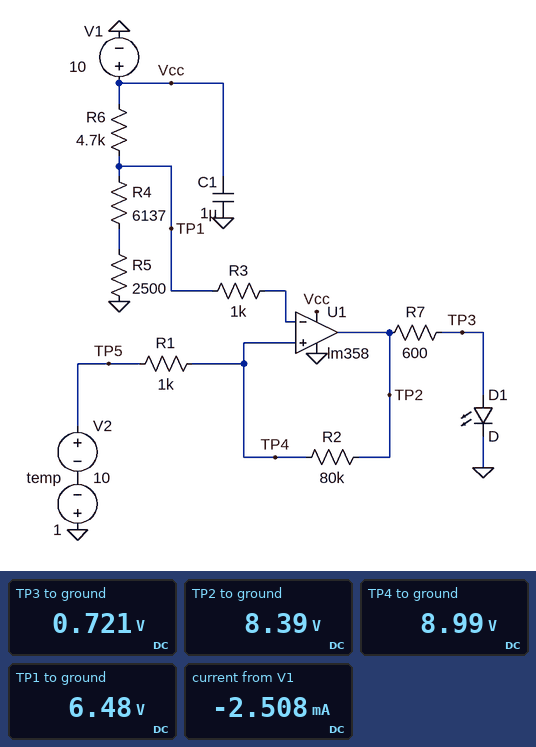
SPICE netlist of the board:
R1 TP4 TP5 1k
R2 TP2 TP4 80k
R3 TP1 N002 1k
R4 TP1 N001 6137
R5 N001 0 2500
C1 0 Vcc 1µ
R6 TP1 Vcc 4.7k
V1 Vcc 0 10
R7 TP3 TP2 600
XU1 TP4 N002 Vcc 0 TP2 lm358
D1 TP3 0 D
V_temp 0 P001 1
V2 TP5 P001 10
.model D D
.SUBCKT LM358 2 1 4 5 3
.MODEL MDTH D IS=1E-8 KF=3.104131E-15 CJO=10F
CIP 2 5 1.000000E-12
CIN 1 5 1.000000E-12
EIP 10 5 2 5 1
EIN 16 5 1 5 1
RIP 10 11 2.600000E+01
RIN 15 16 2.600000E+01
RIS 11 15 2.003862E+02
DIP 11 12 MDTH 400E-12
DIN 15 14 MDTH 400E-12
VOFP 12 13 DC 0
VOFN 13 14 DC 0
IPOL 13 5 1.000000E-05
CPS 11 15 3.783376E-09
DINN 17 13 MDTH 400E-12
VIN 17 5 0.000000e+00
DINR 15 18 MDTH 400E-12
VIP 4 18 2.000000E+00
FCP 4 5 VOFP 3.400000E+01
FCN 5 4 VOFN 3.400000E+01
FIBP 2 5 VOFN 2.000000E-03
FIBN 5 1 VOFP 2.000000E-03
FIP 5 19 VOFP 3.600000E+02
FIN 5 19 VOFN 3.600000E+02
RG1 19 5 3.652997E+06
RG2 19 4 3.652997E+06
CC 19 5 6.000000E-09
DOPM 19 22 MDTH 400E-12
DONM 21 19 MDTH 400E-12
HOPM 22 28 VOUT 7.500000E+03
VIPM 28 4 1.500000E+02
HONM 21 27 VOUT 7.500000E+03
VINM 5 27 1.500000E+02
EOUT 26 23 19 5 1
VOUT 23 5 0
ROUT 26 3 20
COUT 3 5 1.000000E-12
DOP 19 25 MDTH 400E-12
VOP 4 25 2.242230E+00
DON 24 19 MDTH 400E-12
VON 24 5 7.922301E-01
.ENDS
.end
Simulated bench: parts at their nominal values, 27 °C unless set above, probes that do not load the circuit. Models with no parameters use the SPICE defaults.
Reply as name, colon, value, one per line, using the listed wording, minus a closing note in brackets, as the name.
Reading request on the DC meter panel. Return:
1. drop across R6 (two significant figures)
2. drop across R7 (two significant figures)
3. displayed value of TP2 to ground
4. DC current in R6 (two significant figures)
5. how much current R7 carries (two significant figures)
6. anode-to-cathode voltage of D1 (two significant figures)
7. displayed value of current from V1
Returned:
drop across R6: 3.5 V
drop across R7: 7.7 V
displayed value of TP2 to ground: 8.39 V
DC current in R6: 750 µA
how much current R7 carries: 13 mA
anode-to-cathode voltage of D1: 720 mV
displayed value of current from V1: -2.508 mA
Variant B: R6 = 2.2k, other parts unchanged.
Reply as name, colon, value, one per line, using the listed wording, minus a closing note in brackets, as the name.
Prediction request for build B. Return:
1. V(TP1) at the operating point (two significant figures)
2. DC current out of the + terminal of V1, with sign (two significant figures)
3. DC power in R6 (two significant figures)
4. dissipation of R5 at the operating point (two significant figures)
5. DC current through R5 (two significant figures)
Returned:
V(TP1) at the operating point: 8.0 V
DC current out of the + terminal of V1, with sign: -2.3 mA
DC power in R6: 1.9 mW
dissipation of R5 at the operating point: 2.1 mW
DC current through R5: 920 µA
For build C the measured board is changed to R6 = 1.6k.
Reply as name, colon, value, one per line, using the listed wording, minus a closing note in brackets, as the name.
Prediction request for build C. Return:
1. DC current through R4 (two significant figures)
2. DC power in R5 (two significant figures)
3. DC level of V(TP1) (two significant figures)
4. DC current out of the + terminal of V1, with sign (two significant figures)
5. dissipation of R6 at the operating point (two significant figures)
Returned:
DC current through R4: 980 µA
DC power in R5: 2.4 mW
DC level of V(TP1): 8.4 V
DC current out of the + terminal of V1, with sign: -2.3 mA
dissipation of R6 at the operating point: 1.5 mW
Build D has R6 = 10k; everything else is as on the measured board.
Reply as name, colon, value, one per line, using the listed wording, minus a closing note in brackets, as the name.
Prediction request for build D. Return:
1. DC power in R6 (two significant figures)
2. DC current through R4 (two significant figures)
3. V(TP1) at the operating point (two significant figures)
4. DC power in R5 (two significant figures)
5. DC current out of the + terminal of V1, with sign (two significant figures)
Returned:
DC power in R6: 2.9 mW
DC current through R4: 540 µA
V(TP1) at the operating point: 4.6 V
DC power in R5: 720 µW
DC current out of the + terminal of V1, with sign: -2.7 mA
